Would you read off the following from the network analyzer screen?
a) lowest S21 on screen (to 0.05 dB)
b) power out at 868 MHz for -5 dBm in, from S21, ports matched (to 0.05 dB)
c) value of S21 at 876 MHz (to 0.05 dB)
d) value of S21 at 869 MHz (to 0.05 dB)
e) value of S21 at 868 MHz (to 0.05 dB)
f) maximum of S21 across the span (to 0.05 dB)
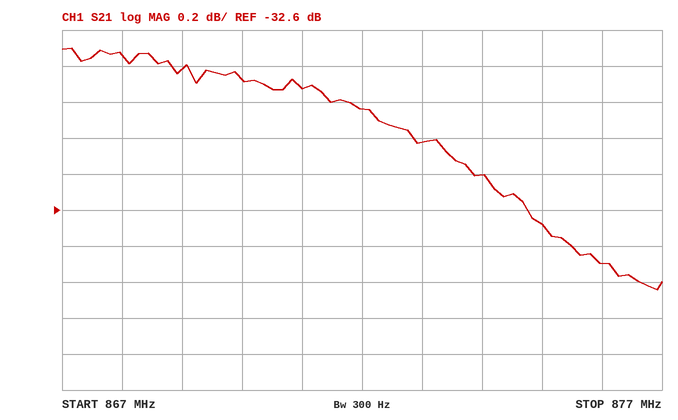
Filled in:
-33.05 dB
-36.75 dBm
-32.90 dB
-31.80 dB
-31.75 dB
-31.70 dB
